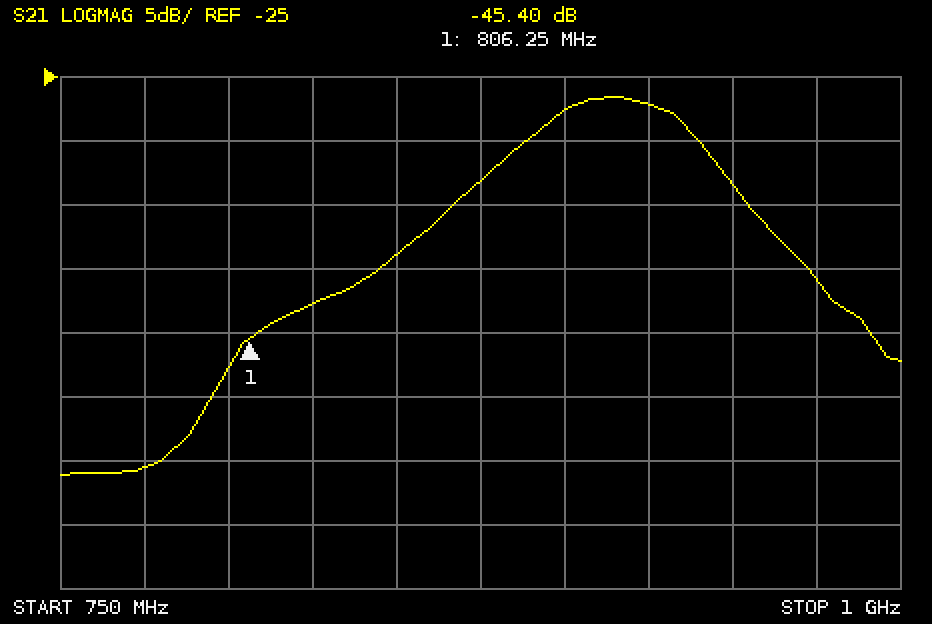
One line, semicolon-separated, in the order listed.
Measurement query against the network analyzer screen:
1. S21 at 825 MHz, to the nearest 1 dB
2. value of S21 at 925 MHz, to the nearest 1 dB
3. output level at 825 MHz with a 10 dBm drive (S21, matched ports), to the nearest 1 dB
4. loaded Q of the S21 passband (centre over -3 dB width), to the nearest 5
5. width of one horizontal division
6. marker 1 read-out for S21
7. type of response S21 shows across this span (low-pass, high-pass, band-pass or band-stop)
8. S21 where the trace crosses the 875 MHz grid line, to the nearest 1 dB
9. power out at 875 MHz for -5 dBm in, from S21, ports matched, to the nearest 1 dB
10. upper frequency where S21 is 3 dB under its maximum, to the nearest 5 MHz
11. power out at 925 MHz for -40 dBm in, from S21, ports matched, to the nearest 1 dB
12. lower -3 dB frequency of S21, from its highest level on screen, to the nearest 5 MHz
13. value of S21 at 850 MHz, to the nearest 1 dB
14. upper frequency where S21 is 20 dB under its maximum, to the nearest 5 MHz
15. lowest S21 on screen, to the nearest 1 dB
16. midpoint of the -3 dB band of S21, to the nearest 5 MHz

-43 dB; -27 dB; -33 dBm; 20; 25 MHz; -45.40 dB; band-pass; -33 dB; -38 dBm; 940 MHz; -67 dBm; 890 MHz; -39 dB; 995 MHz; -56 dB; 915 MHz
